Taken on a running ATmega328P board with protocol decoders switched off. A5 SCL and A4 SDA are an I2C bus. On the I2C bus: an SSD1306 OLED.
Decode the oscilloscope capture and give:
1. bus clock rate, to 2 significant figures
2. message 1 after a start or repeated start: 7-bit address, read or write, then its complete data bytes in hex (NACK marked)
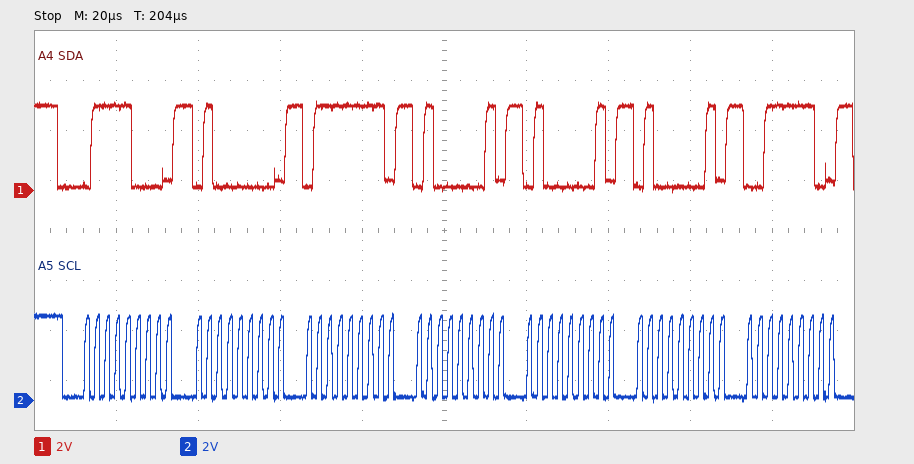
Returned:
400 kHz
0x3C write: 40 7F 41 41 41 3E
